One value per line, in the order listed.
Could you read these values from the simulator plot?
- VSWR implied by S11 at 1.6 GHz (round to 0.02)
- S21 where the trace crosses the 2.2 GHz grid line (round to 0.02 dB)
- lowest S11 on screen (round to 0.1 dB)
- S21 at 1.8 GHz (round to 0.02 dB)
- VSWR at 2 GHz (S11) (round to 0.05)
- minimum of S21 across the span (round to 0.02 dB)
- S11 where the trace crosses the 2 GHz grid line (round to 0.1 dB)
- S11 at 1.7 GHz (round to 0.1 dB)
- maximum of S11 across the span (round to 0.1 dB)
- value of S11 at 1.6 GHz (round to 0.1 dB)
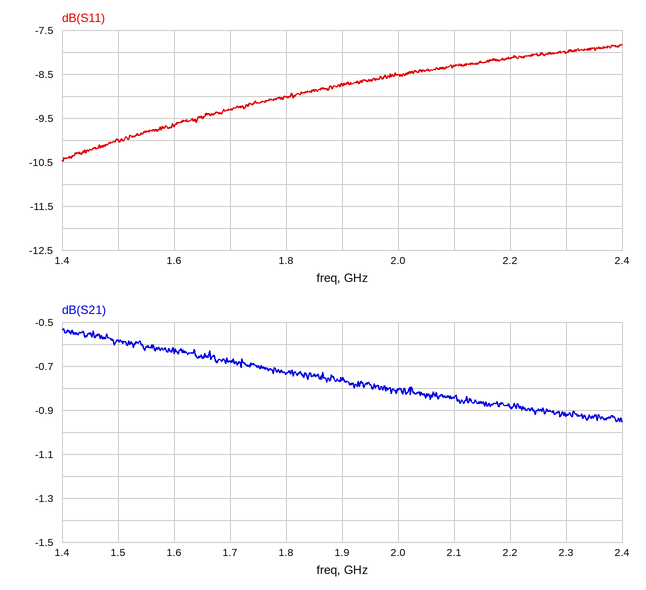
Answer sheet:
1.98
-0.88 dB
-10.5 dB
-0.74 dB
2.20
-0.96 dB
-8.5 dB
-9.3 dB
-7.8 dB
-9.7 dB
